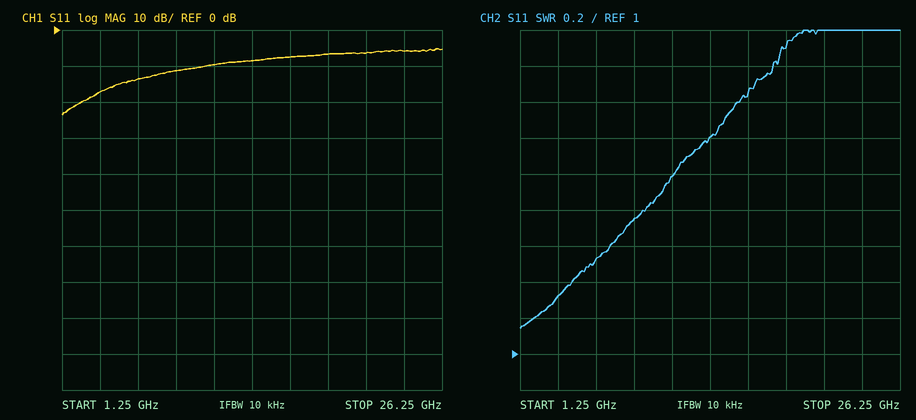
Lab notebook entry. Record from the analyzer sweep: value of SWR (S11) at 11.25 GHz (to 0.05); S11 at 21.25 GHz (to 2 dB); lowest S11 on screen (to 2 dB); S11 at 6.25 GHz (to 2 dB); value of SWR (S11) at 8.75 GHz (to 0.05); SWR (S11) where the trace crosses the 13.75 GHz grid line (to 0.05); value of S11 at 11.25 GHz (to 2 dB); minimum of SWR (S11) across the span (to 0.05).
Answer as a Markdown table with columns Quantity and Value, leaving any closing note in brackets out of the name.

| Quantity | Value |
|---|---|
| value of SWR (S11) at 11.25 GHz | 2.00 |
| S11 at 21.25 GHz | -6 dB |
| lowest S11 on screen | -24 dB |
| S11 at 6.25 GHz | -14 dB |
| value of SWR (S11) at 8.75 GHz | 1.75 |
| SWR (S11) where the trace crosses the 13.75 GHz grid line | 2.20 |
| value of S11 at 11.25 GHz | -10 dB |
| minimum of SWR (S11) across the span | 1.15 |
